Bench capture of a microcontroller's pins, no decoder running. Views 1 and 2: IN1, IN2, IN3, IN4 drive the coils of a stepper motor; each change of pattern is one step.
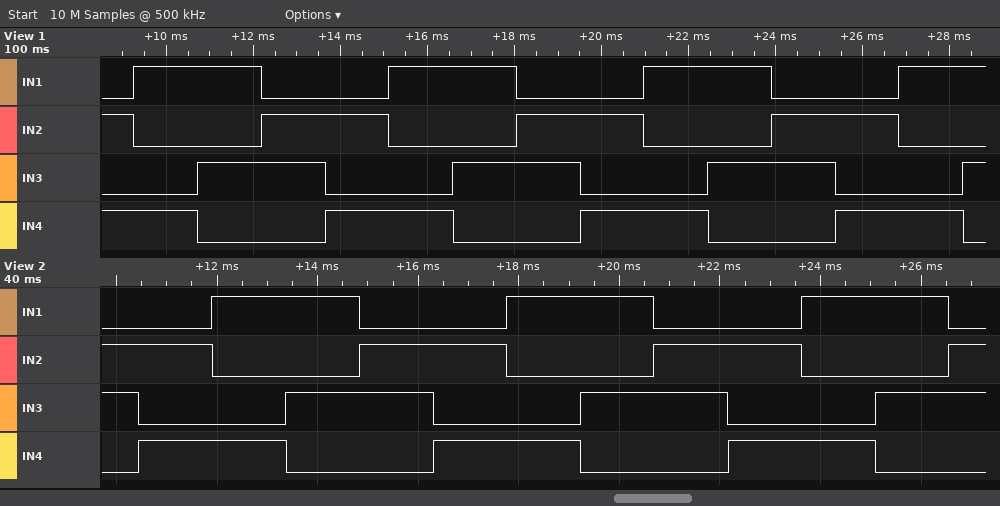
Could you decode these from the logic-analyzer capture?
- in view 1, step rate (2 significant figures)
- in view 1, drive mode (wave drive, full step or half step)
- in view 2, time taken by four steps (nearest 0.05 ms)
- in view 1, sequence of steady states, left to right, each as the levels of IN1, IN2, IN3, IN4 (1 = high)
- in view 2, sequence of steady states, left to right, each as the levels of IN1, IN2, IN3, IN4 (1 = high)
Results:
680 steps/s
full step
5.85 ms
0101 1001 1010 0110 0101 1001 1010 0110 0101 1001 1010 0110 0101 1001 1010
0110 0101 1001 1010 0110 0101 1001 1010 0110 0101 1001 1010 0110
